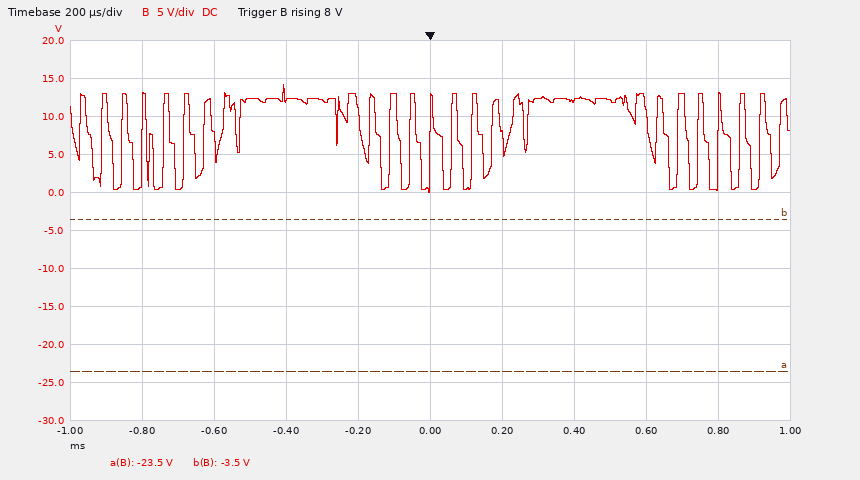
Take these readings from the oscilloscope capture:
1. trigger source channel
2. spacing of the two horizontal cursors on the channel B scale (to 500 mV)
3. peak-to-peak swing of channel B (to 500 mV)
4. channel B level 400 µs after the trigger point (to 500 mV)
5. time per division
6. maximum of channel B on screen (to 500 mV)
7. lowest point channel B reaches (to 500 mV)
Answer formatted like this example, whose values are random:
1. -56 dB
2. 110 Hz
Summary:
1. channel B
2. 20.0 V
3. 14.0 V
4. 12.0 V
5. 200 µs
6. 14.0 V
7. 0.0 V
